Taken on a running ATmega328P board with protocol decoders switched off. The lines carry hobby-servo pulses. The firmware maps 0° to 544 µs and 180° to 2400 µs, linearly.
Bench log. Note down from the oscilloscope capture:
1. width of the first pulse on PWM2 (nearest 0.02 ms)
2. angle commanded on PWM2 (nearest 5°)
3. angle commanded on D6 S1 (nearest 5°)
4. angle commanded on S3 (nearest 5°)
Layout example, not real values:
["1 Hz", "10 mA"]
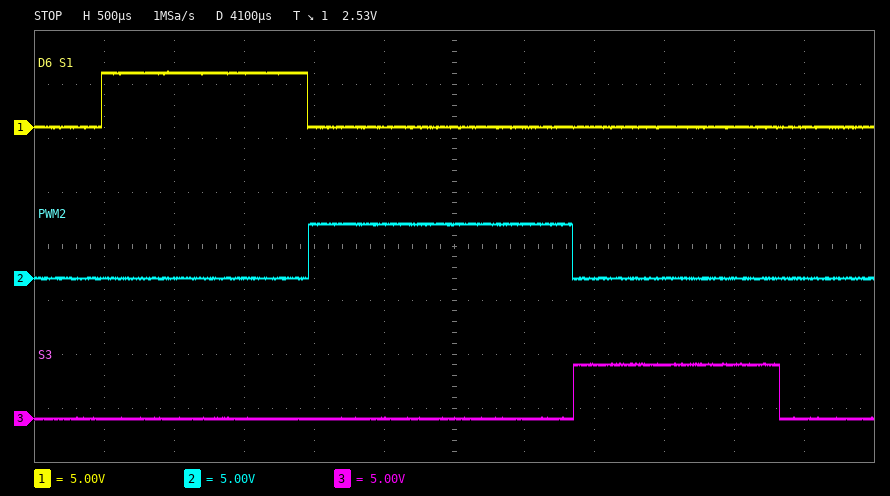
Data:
["1.88 ms", "130°", "90°", "90°"]
